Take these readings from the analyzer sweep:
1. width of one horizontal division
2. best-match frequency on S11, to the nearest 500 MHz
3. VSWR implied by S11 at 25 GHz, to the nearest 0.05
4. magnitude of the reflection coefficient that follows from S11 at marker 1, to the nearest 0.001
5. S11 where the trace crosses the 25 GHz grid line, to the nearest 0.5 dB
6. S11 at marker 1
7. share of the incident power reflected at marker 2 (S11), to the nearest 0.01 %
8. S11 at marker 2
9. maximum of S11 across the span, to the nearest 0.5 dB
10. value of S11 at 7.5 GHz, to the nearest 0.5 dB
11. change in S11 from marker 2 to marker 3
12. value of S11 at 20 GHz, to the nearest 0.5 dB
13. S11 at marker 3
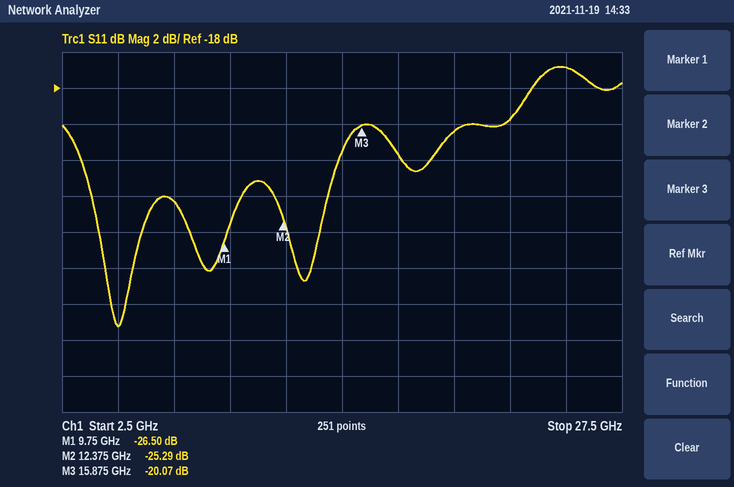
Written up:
2.5 GHz
5.0 GHz
1.35
0.047
-17.0 dB
-26.50 dB
0.30 %
-25.29 dB
-17.0 dB
-24.5 dB
5.22 dB
-20.5 dB
-20.07 dB
